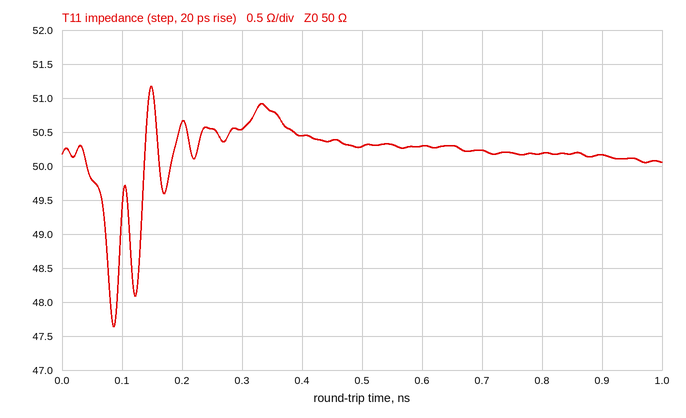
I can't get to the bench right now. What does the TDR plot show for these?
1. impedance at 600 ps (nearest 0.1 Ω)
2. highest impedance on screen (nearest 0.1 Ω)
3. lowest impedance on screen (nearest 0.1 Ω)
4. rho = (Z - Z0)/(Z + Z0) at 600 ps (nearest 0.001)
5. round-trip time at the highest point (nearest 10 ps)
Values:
50.3 Ω
51.2 Ω
47.6 Ω
+0.003
150 ps
